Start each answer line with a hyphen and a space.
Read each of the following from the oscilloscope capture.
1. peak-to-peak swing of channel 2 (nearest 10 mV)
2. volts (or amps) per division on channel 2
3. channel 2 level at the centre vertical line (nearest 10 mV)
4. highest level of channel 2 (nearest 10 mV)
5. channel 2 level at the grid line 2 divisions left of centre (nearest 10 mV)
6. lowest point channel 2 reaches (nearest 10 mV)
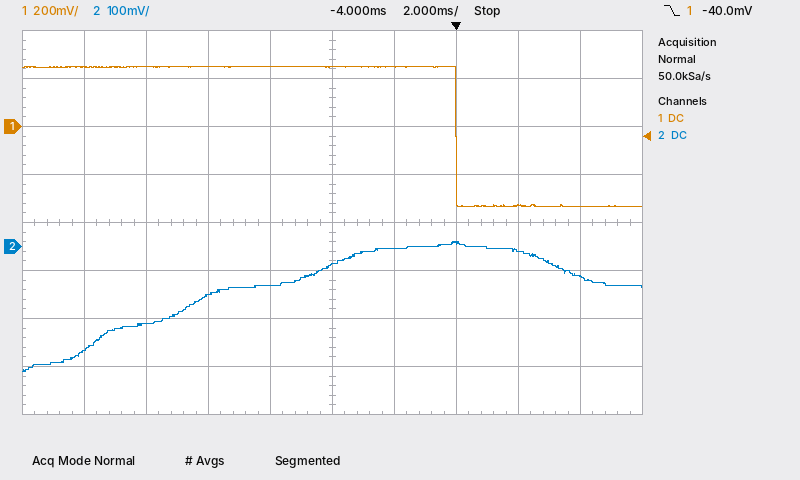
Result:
- 270 mV
- 100 mV
- -40 mV
- 10 mV
- -100 mV
- -260 mV
